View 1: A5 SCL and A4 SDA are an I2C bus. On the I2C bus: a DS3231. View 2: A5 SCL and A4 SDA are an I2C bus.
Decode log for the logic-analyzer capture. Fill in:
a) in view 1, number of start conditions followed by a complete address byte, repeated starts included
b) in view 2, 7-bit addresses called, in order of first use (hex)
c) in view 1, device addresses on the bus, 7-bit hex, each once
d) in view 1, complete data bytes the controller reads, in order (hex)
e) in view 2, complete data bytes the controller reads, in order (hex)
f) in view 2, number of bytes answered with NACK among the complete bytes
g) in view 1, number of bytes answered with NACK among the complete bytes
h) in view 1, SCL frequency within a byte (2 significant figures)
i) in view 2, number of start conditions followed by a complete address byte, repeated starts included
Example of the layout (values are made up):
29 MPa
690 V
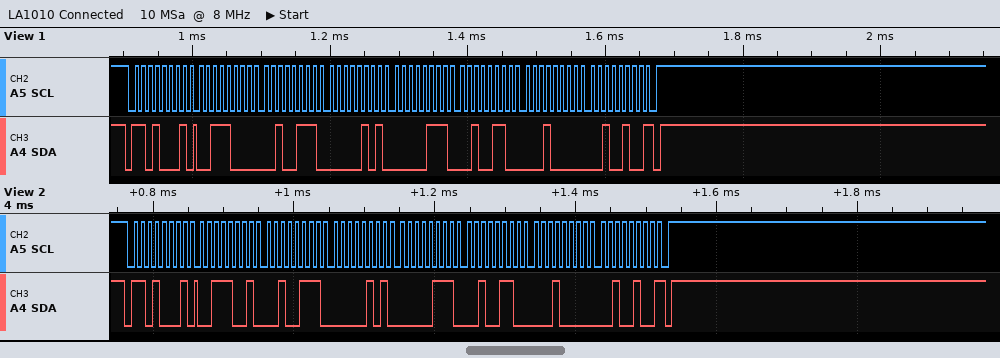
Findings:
1
0x68
0x68
38 27 05 07 26 10 24
39 27 05 07 26 10 24
1
1
100 kHz
1
